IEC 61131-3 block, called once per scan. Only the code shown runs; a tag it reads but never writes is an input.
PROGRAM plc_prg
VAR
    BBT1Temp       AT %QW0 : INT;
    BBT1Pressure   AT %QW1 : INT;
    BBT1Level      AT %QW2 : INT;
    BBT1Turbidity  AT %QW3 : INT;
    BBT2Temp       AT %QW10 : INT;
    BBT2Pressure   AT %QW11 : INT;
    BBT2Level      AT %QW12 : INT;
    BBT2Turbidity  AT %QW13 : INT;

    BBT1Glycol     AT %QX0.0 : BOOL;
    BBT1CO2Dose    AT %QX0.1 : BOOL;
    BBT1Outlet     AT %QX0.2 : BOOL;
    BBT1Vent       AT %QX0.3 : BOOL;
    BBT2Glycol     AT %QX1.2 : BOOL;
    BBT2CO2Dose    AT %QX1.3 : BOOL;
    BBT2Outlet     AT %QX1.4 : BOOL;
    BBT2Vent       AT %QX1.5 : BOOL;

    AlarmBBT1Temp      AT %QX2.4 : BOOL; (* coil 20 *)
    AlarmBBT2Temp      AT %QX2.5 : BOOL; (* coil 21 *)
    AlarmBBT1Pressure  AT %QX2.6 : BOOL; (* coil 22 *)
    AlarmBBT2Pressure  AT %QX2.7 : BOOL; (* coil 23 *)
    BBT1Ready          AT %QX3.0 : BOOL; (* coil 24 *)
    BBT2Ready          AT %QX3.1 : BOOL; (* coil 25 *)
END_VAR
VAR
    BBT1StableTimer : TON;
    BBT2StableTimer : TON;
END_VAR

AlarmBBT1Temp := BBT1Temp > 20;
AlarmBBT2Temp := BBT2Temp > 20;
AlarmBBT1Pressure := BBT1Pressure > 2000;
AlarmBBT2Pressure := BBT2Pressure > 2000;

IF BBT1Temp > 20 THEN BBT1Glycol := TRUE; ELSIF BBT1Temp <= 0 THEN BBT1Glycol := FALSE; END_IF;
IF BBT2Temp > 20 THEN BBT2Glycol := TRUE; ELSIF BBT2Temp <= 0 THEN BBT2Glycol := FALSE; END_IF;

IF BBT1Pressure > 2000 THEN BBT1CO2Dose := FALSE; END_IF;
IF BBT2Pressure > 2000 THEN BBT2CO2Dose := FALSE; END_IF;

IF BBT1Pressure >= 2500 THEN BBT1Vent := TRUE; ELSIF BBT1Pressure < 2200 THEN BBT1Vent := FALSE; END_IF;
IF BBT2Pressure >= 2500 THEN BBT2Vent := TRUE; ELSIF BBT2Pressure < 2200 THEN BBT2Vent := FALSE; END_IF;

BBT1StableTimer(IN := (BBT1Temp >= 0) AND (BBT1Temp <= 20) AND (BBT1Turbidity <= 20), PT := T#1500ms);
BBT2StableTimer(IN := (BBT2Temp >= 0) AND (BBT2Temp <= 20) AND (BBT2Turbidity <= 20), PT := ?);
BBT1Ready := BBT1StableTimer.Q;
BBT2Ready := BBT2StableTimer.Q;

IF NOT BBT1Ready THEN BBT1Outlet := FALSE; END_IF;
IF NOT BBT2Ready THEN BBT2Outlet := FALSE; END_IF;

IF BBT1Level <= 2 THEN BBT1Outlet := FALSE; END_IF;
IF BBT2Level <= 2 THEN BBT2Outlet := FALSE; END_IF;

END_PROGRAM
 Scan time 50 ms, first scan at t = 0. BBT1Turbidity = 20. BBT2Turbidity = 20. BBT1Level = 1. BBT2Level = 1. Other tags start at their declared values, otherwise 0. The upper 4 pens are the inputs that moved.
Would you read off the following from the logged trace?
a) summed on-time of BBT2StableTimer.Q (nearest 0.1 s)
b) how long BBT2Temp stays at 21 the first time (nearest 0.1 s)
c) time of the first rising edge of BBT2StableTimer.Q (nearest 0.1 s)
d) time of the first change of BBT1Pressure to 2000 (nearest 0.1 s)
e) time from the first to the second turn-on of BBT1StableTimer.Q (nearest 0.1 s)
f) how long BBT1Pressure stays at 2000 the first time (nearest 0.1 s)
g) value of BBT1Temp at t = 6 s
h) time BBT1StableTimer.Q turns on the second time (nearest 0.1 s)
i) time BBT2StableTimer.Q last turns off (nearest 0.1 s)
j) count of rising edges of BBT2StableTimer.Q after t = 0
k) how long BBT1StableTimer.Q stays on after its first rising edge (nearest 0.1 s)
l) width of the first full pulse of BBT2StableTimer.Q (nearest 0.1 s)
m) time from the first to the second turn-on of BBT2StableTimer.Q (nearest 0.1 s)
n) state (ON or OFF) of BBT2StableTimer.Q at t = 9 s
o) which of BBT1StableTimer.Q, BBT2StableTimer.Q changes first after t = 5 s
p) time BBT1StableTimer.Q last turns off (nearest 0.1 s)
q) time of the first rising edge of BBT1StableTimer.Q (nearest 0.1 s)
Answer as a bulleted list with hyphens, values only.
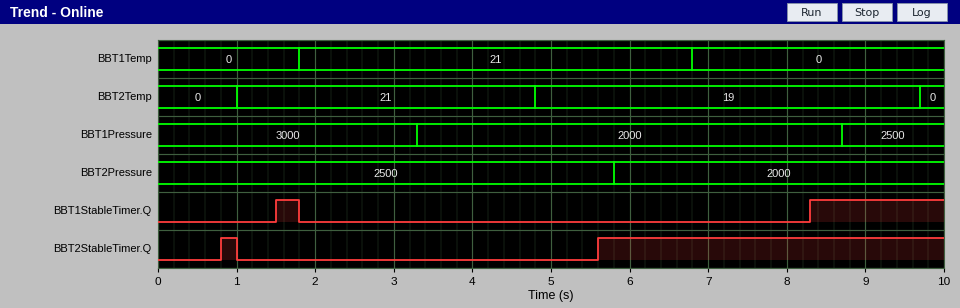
- 4.6 s
- 3.8 s
- 0.8 s
- 3.3 s
- 6.8 s
- 5.4 s
- 21
- 8.3 s
- 1.0 s
- 2
- 0.3 s
- 0.2 s
- 4.8 s
- ON
- BBT2StableTimer.Q
- 1.8 s
- 1.5 s
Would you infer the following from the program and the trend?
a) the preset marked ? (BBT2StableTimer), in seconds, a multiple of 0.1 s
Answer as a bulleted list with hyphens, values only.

- 0.8 s
